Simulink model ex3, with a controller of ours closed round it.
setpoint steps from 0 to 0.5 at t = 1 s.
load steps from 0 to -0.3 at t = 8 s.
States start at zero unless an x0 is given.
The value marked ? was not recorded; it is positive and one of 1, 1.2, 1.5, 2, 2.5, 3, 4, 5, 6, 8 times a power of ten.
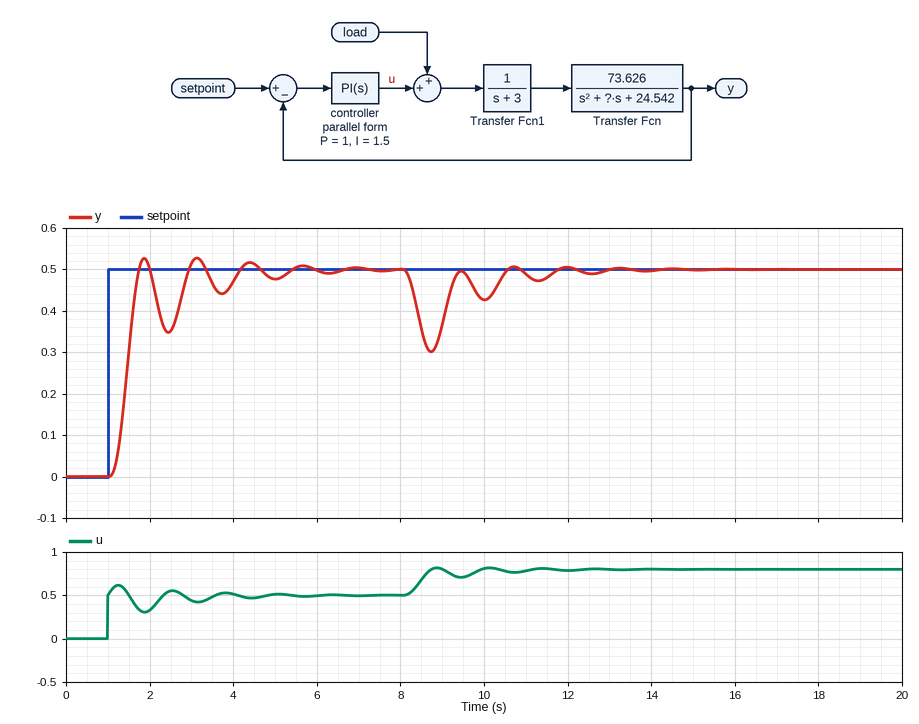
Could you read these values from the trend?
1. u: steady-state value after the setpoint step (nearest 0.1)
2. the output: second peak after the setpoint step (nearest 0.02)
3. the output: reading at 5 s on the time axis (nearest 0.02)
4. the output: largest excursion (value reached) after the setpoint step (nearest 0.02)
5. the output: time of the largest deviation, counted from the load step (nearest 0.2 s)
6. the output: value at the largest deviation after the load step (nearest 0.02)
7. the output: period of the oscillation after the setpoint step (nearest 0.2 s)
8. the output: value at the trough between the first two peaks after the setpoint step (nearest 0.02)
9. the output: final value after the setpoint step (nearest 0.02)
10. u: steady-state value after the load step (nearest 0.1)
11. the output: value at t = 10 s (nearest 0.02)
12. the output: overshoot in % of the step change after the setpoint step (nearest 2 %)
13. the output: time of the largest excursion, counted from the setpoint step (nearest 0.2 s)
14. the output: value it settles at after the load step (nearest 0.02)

0.5
0.52
0.48
0.52
0.8 s
0.30
1.2 s
0.34
0.50
0.8
0.42
6 %
2.2 s
0.50
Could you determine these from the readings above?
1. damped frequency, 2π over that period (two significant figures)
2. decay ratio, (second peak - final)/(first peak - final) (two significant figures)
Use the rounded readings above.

5.2 rad/s
1.0
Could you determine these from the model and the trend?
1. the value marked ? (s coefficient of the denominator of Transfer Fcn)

4
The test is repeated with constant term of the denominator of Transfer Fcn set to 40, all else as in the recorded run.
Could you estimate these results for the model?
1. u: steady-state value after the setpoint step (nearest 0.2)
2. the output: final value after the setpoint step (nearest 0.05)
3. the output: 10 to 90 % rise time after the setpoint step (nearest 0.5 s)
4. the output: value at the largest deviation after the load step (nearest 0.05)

0.8
0.50
2.5 s
0.35
